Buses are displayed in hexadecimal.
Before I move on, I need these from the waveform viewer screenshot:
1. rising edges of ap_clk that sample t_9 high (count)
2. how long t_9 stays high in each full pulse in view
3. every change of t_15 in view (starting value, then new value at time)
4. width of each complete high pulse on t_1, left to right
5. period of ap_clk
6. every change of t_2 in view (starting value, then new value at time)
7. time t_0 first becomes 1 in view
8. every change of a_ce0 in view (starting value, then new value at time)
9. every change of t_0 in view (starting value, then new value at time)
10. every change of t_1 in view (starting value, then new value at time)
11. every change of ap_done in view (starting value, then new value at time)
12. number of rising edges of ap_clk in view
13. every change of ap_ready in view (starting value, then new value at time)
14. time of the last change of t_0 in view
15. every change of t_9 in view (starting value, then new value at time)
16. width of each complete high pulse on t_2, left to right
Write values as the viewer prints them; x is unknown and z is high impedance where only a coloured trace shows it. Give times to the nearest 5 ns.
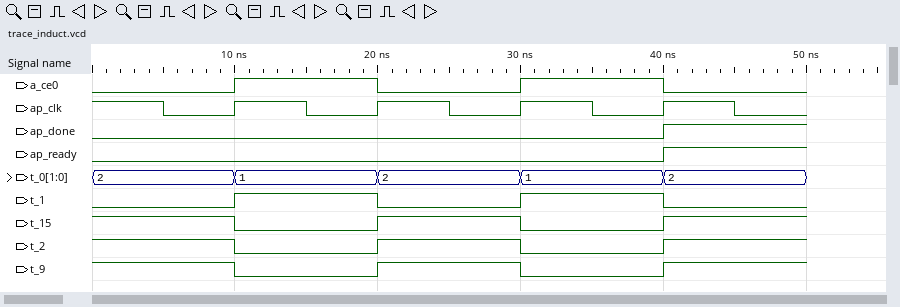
2
10 ns
1, 0 at 10 ns, 1 at 20 ns, 0 at 30 ns, 1 at 40 ns
10 ns, 10 ns
10 ns
1, 0 at 10 ns, 1 at 20 ns, 0 at 30 ns, 1 at 40 ns
10 ns
0, 1 at 10 ns, 0 at 20 ns, 1 at 30 ns, 0 at 40 ns
2, 1 at 10 ns, 2 at 20 ns, 1 at 30 ns, 2 at 40 ns
0, 1 at 10 ns, 0 at 20 ns, 1 at 30 ns, 0 at 40 ns
0, 1 at 40 ns
4
0, 1 at 40 ns
40 ns
1, 0 at 10 ns, 1 at 20 ns, 0 at 30 ns, 1 at 40 ns
10 ns
